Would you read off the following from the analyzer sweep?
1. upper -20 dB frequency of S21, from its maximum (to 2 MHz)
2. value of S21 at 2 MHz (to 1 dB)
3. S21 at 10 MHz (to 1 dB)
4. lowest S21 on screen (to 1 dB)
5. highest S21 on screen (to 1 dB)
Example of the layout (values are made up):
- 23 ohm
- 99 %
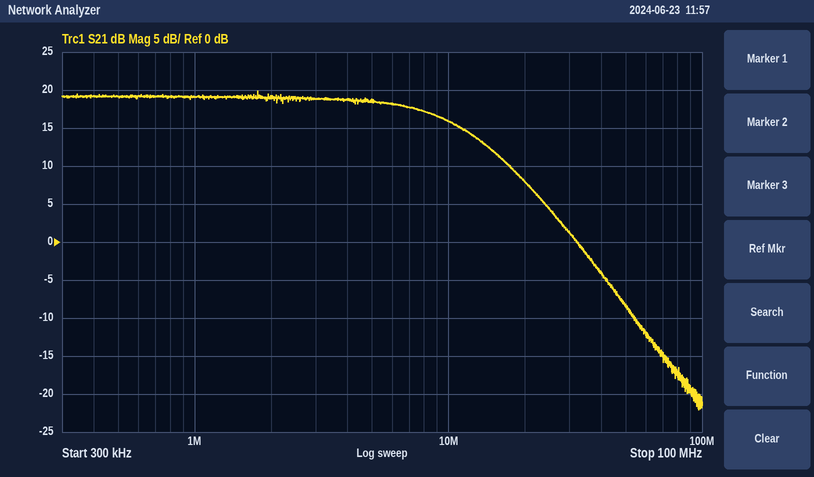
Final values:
- 32 MHz
- 19 dB
- 16 dB
- -22 dB
- 20 dB
